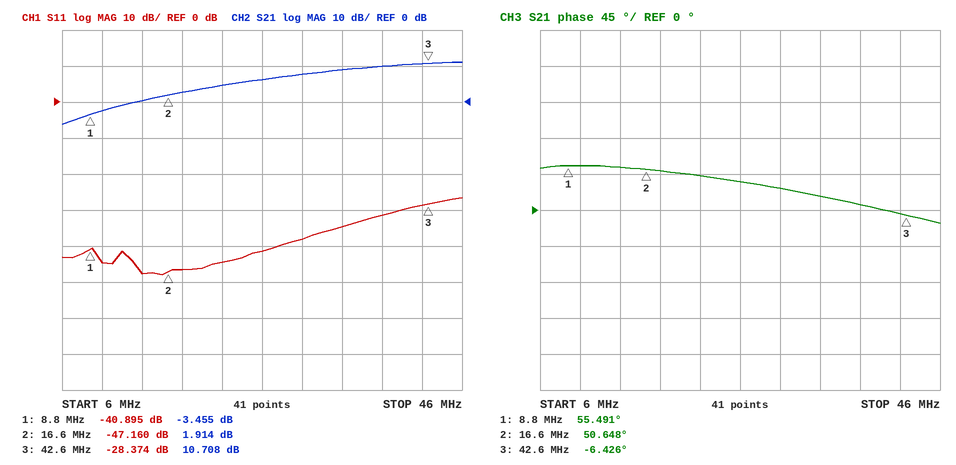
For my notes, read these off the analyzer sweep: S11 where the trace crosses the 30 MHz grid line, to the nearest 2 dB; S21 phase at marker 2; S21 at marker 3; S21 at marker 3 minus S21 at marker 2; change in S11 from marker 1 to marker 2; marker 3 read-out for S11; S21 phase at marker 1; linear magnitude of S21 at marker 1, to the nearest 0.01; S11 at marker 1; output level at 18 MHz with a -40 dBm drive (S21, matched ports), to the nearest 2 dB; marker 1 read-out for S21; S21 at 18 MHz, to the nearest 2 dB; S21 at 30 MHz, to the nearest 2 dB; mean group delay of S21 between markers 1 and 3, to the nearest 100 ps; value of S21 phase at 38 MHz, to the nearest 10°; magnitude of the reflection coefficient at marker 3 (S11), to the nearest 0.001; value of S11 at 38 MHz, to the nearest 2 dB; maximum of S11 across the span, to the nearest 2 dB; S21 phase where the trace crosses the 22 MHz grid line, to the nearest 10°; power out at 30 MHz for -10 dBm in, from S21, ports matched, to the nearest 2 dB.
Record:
-38 dB
50.648°
10.708 dB
8.794 dB
-6.265 dB
-28.374 dB
55.491°
0.67
-40.895 dB
-38 dBm
-3.455 dB
2 dB
8 dB
5.1 ns
10°
0.038
-32 dB
-26 dB
40°
-2 dBm
